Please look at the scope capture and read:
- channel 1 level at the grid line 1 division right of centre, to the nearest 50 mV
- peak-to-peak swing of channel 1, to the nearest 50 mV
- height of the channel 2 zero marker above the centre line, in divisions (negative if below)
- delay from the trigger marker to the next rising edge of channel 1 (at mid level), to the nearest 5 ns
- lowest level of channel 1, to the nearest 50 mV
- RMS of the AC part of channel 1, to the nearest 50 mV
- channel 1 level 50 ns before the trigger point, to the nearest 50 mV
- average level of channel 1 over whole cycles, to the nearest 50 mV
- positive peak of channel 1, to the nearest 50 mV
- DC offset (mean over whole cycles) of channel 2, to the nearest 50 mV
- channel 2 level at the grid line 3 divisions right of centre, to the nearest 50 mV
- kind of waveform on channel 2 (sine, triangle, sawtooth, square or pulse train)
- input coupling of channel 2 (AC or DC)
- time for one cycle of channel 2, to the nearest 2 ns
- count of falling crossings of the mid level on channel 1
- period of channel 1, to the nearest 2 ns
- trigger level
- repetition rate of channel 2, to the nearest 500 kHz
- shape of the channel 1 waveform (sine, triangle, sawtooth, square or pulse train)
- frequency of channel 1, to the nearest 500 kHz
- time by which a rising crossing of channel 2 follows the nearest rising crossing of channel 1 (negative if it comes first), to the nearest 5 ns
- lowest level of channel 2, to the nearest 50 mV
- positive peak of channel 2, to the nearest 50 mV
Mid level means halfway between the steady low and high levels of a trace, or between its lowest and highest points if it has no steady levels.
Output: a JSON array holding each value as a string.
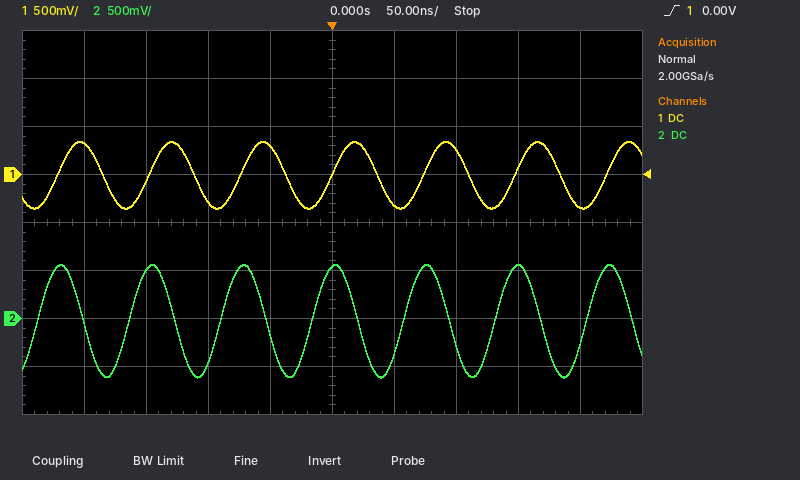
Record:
["-300 mV", "700 mV", "-2.0 div", "75 ns", "-350 mV", "250 mV", "300 mV", "0 mV", "350 mV", "0 mV", "550 mV", "sine", "DC", "74 ns", "6", "74 ns", "0.00 V", "13.5 MHz", "sine", "13.5 MHz", "-15 ns", "-600 mV", "550 mV"]
